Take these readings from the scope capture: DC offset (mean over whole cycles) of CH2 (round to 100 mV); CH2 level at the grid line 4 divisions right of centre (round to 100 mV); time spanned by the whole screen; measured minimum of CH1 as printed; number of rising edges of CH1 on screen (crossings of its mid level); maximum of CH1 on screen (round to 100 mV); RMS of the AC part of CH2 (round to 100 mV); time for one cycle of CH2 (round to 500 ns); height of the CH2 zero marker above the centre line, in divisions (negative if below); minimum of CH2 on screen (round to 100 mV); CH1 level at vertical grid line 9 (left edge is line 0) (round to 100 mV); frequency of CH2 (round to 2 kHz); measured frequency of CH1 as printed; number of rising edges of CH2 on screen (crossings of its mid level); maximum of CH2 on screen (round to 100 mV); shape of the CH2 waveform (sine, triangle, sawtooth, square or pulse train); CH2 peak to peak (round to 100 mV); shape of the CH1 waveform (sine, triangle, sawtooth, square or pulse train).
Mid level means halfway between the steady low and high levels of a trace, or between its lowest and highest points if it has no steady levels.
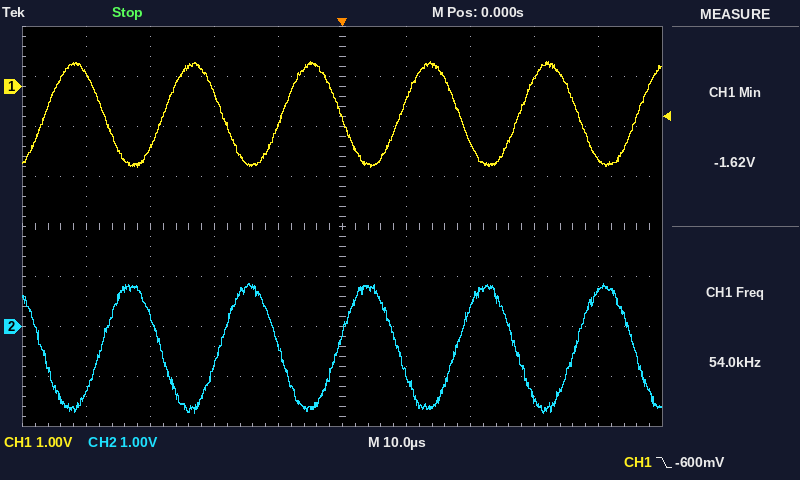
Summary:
-400 mV
700 mV
100 µs
-1.62 V
6
500 mV
900 mV
18.5 µs
-2.0 div
-1.7 V
-1.4 V
54 kHz
54.0 kHz
5
900 mV
sine
2.6 V
sine
